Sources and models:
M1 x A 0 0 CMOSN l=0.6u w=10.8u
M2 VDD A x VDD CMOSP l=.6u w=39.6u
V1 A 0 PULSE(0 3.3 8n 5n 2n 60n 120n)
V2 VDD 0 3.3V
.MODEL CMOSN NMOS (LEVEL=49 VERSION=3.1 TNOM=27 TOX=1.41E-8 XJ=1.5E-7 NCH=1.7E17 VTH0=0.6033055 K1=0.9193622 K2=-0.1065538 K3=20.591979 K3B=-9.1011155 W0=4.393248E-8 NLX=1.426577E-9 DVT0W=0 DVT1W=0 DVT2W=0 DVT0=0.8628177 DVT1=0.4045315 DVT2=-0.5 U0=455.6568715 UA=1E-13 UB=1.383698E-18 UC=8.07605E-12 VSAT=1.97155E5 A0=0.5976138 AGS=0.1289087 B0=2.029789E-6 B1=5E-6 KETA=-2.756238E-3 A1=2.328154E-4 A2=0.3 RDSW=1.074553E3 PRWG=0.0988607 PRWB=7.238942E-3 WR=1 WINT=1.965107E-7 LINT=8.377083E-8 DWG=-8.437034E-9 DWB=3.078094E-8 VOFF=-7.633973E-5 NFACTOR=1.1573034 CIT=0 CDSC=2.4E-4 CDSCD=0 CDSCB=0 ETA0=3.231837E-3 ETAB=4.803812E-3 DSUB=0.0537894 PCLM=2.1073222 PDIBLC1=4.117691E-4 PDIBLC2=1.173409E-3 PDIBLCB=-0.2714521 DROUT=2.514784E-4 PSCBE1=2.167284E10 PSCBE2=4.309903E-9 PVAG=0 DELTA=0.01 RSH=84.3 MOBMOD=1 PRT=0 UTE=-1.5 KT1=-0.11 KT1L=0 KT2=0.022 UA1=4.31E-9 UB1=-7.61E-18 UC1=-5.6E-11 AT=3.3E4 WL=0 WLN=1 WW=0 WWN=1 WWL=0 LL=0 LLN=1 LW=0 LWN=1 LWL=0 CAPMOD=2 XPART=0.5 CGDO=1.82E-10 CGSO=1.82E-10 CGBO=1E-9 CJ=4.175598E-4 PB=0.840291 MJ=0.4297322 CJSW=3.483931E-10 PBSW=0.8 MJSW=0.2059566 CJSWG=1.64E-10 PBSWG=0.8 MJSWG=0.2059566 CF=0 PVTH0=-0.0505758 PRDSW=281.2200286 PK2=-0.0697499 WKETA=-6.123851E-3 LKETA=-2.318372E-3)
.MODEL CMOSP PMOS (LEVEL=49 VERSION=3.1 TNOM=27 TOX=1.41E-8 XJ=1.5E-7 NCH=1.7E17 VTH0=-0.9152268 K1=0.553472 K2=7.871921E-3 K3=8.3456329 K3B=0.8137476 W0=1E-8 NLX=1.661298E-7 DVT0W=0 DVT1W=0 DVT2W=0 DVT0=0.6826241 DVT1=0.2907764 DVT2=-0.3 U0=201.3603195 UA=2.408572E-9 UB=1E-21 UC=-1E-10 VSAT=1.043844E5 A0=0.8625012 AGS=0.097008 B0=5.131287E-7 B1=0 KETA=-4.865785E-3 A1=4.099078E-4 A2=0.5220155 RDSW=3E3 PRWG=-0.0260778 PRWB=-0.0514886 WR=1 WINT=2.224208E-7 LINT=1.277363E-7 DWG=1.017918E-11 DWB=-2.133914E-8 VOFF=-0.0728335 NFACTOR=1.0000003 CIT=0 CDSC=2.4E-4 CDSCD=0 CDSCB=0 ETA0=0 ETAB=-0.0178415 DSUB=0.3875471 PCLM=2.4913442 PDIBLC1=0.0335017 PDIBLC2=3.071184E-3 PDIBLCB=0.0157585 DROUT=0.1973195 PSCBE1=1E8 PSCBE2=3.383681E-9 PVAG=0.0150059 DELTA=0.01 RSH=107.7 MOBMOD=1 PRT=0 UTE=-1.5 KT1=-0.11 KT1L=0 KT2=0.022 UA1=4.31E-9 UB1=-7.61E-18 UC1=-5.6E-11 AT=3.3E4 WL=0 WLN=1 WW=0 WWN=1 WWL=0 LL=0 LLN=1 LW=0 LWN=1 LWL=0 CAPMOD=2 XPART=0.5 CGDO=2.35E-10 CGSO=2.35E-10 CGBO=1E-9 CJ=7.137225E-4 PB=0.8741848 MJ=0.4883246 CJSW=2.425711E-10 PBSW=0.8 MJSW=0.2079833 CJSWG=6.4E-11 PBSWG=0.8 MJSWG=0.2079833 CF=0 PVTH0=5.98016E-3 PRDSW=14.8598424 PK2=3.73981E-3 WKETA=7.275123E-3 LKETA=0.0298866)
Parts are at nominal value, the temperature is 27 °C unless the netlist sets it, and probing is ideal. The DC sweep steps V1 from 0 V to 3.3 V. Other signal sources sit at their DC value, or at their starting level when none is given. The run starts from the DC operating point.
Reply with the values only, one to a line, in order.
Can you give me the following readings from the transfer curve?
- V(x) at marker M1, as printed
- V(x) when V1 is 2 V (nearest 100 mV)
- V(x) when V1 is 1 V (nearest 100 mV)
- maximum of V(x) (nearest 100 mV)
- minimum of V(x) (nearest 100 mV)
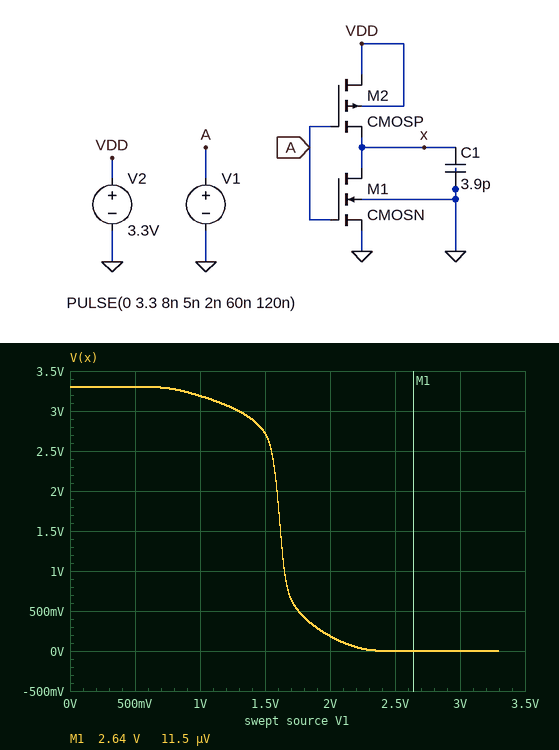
11.5 µV
200 mV
3.2 V
3.3 V
0 V
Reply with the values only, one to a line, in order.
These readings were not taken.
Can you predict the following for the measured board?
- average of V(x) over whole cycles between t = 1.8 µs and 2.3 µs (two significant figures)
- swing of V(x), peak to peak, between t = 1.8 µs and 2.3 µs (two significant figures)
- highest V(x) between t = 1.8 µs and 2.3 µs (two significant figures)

1.6 V
3.3 V
3.3 V
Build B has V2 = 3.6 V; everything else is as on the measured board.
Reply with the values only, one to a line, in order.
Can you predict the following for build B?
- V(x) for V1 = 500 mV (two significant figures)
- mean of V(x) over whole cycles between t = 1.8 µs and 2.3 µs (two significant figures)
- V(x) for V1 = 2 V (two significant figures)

3.6 V
1.7 V
510 mV
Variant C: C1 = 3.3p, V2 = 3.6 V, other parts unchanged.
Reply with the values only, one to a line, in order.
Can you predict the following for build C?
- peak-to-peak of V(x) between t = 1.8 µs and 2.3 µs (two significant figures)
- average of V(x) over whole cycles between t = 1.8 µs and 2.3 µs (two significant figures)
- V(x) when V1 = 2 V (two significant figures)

3.6 V
1.7 V
510 mV
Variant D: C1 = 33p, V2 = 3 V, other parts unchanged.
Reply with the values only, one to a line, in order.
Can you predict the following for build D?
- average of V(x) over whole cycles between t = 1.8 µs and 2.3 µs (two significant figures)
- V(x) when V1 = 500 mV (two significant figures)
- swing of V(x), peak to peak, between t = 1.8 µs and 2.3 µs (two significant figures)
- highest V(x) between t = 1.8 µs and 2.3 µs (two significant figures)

1.5 V
3.0 V
2.8 V
2.9 V
